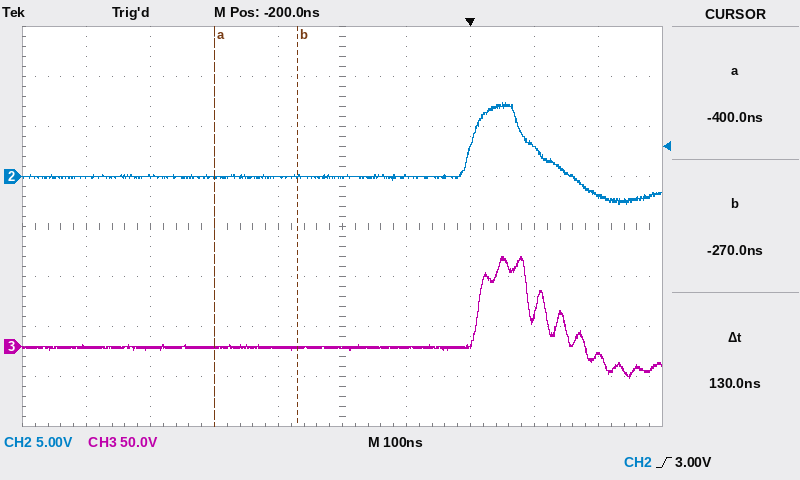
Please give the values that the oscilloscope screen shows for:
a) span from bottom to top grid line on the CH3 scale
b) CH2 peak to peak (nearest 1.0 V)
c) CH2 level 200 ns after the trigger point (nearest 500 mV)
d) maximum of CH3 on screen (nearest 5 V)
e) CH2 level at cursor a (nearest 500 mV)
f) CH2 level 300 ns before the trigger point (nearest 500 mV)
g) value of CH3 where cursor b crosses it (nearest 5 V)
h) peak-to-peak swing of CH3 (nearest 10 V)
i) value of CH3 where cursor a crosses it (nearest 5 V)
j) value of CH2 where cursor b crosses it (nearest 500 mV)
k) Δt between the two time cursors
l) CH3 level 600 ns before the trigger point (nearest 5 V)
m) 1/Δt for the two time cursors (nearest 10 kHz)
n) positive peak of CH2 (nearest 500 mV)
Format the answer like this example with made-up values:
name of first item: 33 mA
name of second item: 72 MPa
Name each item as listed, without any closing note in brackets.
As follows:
span from bottom to top grid line on the CH3 scale: 400 V
CH2 peak to peak: 10.0 V
CH2 level 200 ns after the trigger point: -2.0 V
maximum of CH3 on screen: 90 V
CH2 level at cursor a: 0.0 V
CH2 level 300 ns before the trigger point: 0.0 V
value of CH3 where cursor b crosses it: 0 V
peak-to-peak swing of CH3: 120 V
value of CH3 where cursor a crosses it: 0 V
value of CH2 where cursor b crosses it: 0.0 V
Δt between the two time cursors: 130 ns
CH3 level 600 ns before the trigger point: 0 V
1/Δt for the two time cursors: 7.69 MHz
positive peak of CH2: 7.5 V
